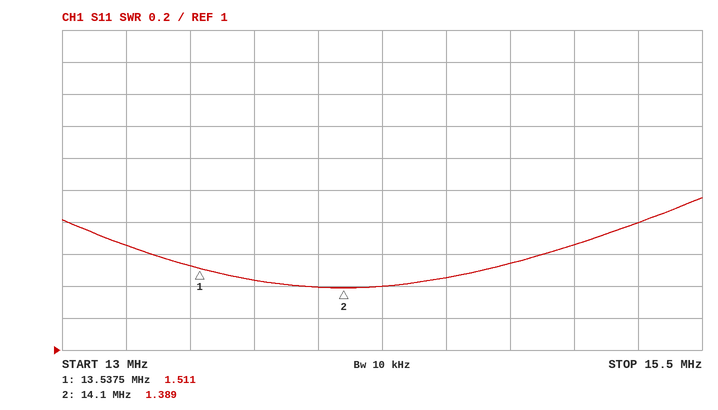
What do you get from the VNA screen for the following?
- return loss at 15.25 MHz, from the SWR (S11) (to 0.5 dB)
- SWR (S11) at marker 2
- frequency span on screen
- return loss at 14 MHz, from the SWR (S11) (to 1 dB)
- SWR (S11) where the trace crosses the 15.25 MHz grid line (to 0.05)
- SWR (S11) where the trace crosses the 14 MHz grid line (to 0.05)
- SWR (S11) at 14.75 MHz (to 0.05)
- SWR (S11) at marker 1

11.0 dB
1.389
2.5 MHz
16 dB
1.80
1.40
1.55
1.511
